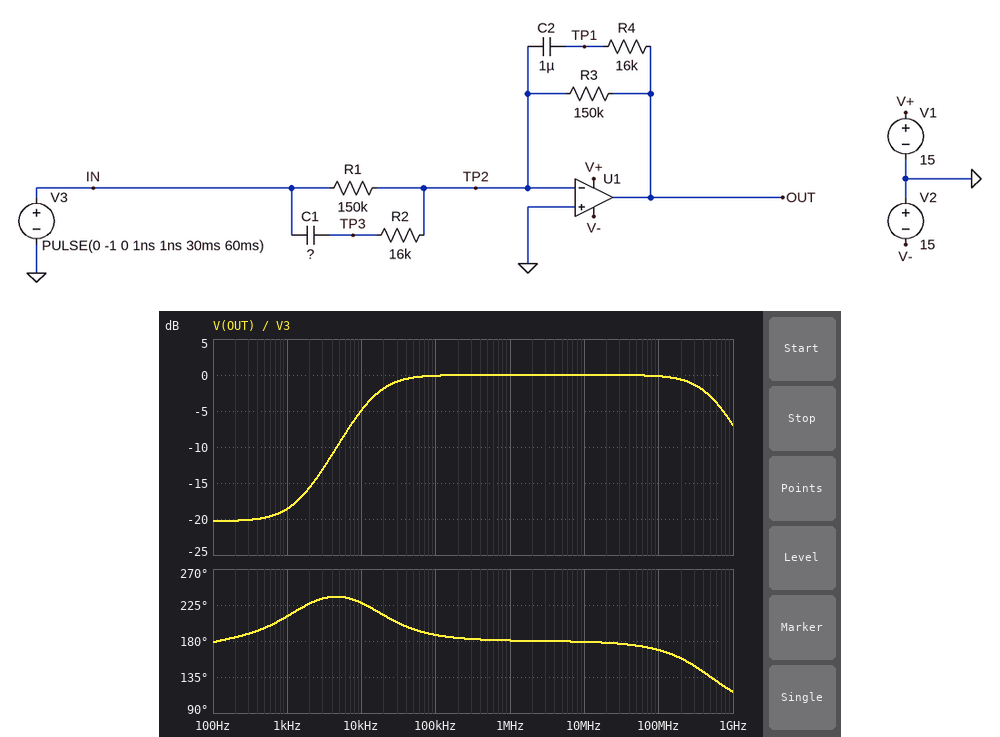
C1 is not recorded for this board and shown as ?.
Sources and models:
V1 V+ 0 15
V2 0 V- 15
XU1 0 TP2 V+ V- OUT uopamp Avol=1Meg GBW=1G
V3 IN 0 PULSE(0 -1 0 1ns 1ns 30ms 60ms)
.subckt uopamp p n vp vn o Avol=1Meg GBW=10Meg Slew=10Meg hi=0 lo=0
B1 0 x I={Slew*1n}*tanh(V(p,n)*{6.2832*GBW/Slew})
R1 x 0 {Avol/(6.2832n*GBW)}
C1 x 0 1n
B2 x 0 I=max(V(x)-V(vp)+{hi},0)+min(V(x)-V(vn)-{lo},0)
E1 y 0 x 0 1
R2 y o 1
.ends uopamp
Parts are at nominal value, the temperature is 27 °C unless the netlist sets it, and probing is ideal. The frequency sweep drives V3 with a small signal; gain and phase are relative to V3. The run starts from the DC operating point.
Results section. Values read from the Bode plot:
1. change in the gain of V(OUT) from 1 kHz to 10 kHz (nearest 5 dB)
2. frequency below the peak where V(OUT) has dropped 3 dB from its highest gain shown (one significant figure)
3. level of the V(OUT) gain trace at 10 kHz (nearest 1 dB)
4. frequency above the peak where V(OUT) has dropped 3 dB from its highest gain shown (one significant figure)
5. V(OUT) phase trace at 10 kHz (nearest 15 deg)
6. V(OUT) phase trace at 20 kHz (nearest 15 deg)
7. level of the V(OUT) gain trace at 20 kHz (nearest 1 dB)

15 dB
10 kHz
-5 dB
500 MHz
225 deg
210 deg
-2 dB
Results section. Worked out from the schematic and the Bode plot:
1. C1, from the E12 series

680 pF
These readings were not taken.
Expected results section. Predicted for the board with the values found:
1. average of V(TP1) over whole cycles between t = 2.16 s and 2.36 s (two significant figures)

500 mV
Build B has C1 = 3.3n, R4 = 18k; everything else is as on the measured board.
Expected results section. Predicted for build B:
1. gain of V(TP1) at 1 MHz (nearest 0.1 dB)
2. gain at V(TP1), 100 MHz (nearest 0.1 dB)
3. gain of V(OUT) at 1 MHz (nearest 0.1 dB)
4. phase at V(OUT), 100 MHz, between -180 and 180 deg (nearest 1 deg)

-59.0 dB
-19.3 dB
0.9 dB
168 deg
